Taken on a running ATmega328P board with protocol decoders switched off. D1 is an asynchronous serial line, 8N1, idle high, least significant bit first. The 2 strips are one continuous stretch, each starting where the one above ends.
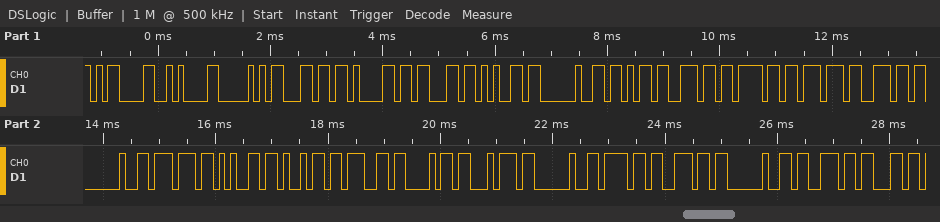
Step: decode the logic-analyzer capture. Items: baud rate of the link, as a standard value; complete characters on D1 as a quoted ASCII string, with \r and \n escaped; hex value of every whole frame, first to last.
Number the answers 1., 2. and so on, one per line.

1. 9600 baud
2. "\r\nPlace known weight on sc"
3. 0x0D 0x0A 0x50 0x6C 0x61 0x63 0x65 0x20 0x6B 0x6E 0x6F 0x77 0x6E 0x20 0x77 0x65 0x69 0x67 0x68 0x74 0x20 0x6F 0x6E 0x20 0x73 0x63
